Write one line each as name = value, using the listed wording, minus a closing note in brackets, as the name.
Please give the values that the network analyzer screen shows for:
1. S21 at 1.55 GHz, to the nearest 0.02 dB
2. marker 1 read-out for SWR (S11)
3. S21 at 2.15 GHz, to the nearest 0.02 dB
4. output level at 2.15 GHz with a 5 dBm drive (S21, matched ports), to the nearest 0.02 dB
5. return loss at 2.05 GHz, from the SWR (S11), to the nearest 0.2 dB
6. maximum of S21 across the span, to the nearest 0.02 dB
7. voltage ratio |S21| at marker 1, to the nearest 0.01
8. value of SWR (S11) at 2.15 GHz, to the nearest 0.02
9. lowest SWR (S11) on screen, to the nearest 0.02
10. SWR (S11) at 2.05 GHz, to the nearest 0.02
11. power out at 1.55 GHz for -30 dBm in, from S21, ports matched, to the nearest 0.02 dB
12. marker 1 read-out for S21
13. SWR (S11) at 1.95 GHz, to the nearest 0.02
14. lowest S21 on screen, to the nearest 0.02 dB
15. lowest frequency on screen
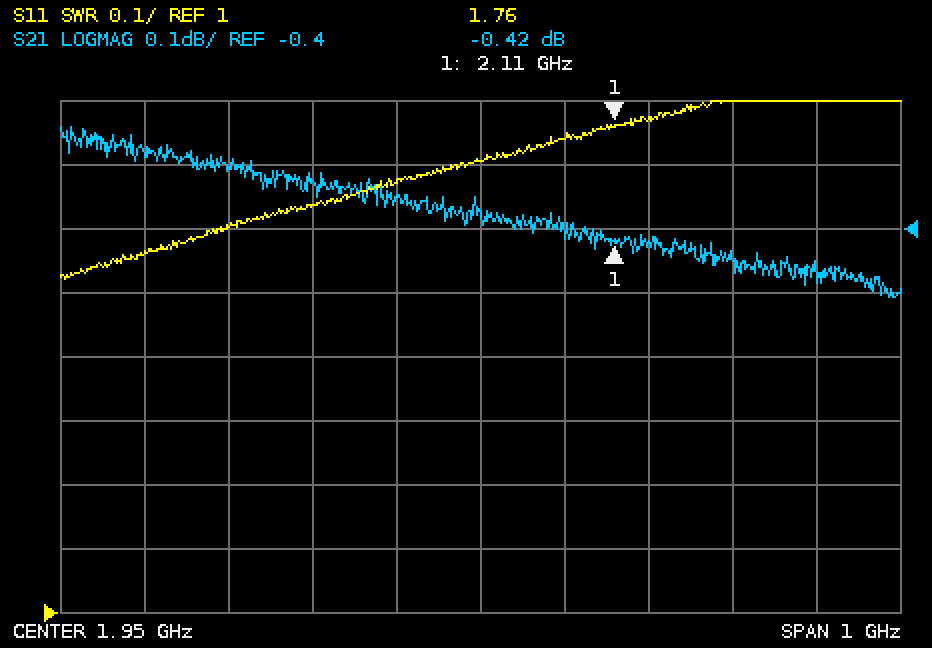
S21 at 1.55 GHz, to the nearest 0.02 dB = -0.28 dB
marker 1 read-out for SWR = 1.76
S21 at 2.15 GHz, to the nearest 0.02 dB = -0.42 dB
output level at 2.15 GHz with a 5 dBm drive (S21, matched ports), to the nearest 0.02 dB = 4.58 dBm
return loss at 2.05 GHz, from the SWR (S11), to the nearest 0.2 dB = 11.4 dB
maximum of S21 across the span, to the nearest 0.02 dB = -0.24 dB
voltage ratio |S21| at marker 1, to the nearest 0.01 = 0.95
value of SWR (S11) at 2.15 GHz, to the nearest 0.02 = 1.78
lowest SWR (S11) on screen, to the nearest 0.02 = 1.52
SWR (S11) at 2.05 GHz, to the nearest 0.02 = 1.74
power out at 1.55 GHz for -30 dBm in, from S21, ports matched, to the nearest 0.02 dB = -30.28 dBm
marker 1 read-out for S21 = -0.42 dB
SWR (S11) at 1.95 GHz, to the nearest 0.02 = 1.70
lowest S21 on screen, to the nearest 0.02 dB = -0.50 dB
lowest frequency on screen = 1.45 GHz
